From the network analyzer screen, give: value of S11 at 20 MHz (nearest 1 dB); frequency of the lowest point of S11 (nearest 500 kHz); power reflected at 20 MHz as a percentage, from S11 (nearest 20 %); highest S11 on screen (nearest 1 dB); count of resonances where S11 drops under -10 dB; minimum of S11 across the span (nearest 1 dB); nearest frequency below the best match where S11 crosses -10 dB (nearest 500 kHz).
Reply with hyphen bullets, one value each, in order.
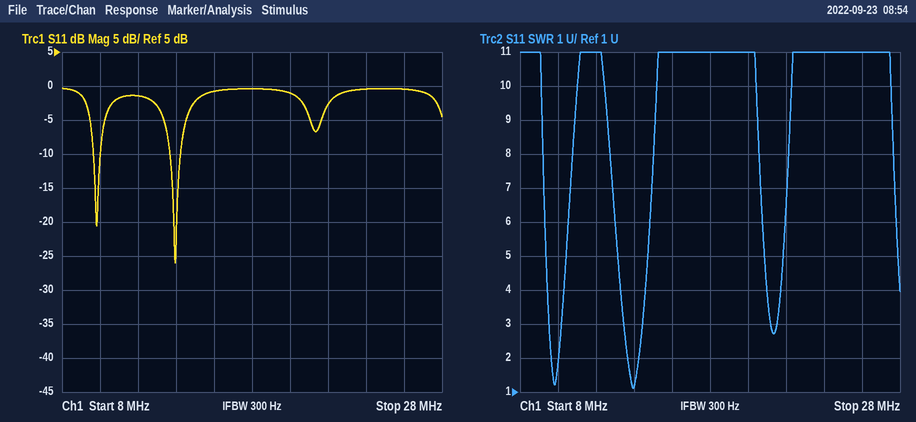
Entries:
- -1 dB
- 14.0 MHz
- 80 %
- 0 dB
- 2
- -26 dB
- 13.5 MHz
